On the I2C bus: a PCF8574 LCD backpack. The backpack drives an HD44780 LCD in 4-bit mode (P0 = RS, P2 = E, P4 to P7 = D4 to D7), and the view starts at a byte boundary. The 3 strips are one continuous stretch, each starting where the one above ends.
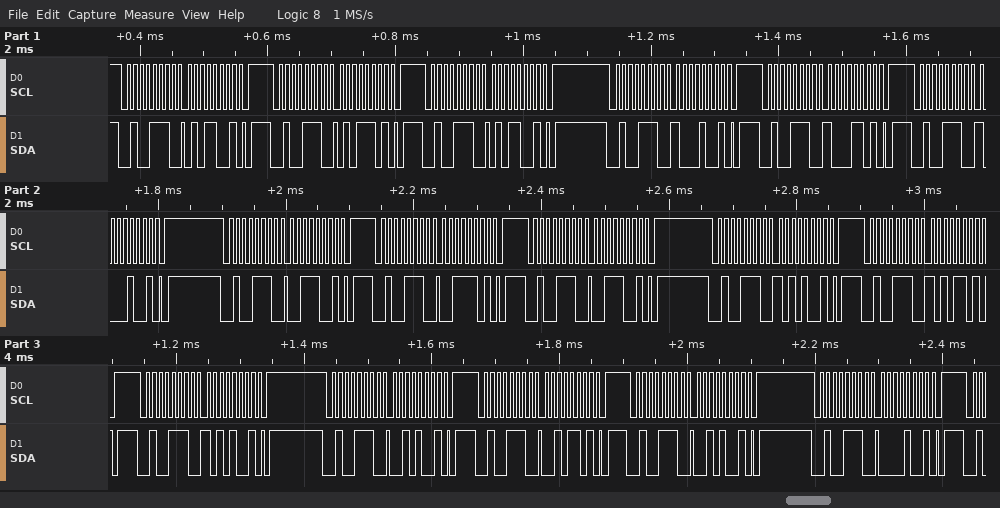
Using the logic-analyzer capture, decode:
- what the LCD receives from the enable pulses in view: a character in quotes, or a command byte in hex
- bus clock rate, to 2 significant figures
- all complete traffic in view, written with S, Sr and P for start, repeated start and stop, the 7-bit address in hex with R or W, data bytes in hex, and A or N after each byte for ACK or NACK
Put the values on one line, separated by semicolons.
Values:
'X' ':'; 100 kHz; S 27W A 59 A P S 27W A 5D A P S 27W A 59 A P S 27W A 89 A P S 27W A 8D A P S 27W A 89 A P S 27W A 39 A P S 27W A 3D A P S 27W A 39 A P S 27W A A9 A P S 27W A AD A P S 27W A A9 A P S 27W A 29 A P S 27W A 2D A P S 27W A 29 A P S 27W A 09 A P
